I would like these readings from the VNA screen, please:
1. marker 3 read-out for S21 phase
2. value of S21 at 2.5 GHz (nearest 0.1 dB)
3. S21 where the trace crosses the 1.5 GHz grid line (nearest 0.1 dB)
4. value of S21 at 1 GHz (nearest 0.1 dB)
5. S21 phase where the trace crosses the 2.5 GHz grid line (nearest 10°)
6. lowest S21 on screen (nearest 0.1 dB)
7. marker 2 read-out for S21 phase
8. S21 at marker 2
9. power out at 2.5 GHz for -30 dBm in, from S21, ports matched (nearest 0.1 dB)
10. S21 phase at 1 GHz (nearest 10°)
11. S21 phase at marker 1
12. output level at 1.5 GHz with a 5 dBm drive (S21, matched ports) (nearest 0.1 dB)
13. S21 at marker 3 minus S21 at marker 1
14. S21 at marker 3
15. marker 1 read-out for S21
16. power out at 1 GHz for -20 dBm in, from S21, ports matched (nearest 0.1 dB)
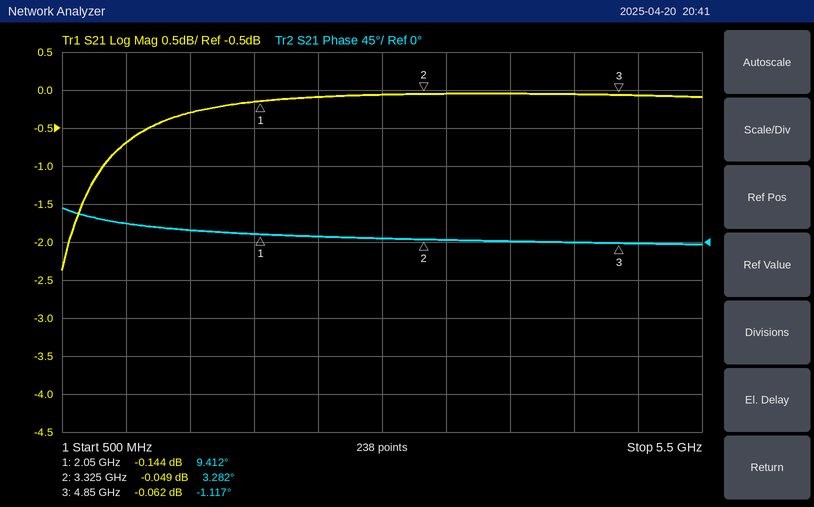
-1.117°
-0.1 dB
-0.3 dB
-0.7 dB
10°
-2.4 dB
3.282°
-0.049 dB
-30.1 dBm
20°
9.412°
4.7 dBm
0.082 dB
-0.062 dB
-0.144 dB
-20.7 dBm
